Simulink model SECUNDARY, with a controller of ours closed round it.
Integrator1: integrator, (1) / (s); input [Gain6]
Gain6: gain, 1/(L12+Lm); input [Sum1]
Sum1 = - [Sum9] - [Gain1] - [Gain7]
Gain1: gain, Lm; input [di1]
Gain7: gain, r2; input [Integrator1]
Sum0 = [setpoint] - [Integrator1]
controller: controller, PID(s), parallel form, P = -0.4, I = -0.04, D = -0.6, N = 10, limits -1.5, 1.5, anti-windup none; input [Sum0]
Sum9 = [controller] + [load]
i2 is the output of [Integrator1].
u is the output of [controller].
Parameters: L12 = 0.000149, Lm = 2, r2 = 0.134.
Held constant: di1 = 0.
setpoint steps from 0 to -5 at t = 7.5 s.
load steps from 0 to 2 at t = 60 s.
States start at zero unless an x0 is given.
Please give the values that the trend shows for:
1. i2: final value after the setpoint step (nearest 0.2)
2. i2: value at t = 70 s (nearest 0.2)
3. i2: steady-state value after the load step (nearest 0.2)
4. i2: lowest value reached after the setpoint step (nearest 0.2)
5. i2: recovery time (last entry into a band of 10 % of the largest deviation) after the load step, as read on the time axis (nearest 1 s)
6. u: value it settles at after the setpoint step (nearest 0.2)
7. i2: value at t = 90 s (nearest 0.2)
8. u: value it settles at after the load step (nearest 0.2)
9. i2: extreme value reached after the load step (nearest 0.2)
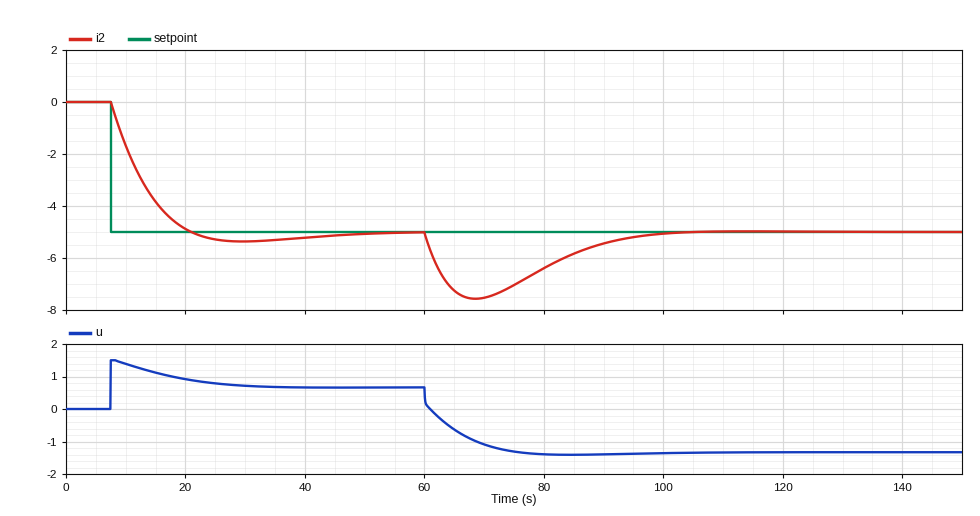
-5.0
-7.6
-5.0
-5.4
94 s
0.6
-5.4
-1.4
-7.6
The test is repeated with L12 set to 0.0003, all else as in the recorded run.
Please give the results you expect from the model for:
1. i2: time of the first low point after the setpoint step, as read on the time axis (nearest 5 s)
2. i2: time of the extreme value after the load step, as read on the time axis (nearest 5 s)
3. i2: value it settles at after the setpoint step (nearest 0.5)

30 s
70 s
-5.0
